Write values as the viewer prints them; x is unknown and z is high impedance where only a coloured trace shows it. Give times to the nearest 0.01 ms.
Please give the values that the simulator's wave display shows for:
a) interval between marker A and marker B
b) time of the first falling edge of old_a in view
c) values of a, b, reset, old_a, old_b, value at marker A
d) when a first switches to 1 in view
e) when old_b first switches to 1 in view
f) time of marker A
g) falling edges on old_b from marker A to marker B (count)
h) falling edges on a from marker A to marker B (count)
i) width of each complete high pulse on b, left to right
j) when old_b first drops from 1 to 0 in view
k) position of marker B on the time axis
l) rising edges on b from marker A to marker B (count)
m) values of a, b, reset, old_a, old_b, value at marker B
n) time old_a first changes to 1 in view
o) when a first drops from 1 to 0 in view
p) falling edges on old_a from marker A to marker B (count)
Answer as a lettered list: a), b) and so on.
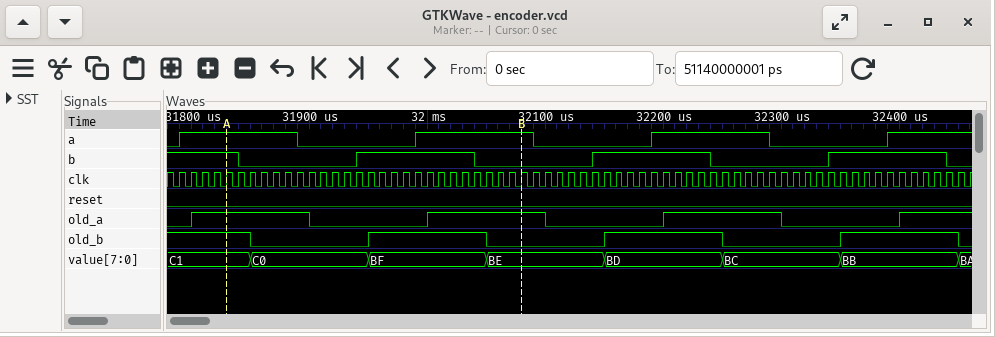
a) 0.25 ms
b) 31.9 ms
c) a=1, b=1, reset=0, old_a=1, old_b=1, value=C1
d) 31.79 ms
e) 31.95 ms
f) 31.83 ms
g) 2
h) 1
i) 0.1 ms, 0.1 ms, 0.1 ms
j) 31.85 ms
k) 32.08 ms
l) 1
m) a=1, b=0, reset=0, old_a=1, old_b=0, value=BE
n) 31.8 ms
o) 31.89 ms
p) 1
